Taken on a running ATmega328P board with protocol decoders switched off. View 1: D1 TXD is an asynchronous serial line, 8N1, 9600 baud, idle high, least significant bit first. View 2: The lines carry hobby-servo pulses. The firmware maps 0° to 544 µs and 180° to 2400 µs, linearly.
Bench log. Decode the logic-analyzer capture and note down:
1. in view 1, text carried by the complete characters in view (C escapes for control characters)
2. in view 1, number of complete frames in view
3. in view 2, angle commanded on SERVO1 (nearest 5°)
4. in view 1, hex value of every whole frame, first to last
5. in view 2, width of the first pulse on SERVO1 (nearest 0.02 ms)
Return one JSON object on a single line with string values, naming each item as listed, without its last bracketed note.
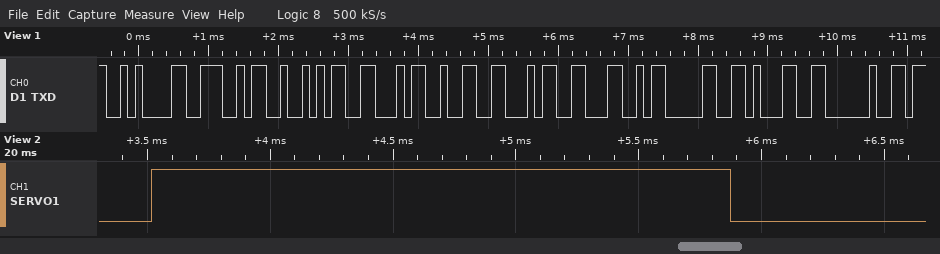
{"in view 1, text carried by the complete characters in view": "\"\\nNRF24L01 \"", "in view 1, number of complete frames in view": "10", "in view 2, angle commanded on SERVO1": "175°", "in view 1, hex value of every whole frame, first to last": "0A 4E 52 46 32 34 4C 30 31 20", "in view 2, width of the first pulse on SERVO1": "2.36 ms"}
